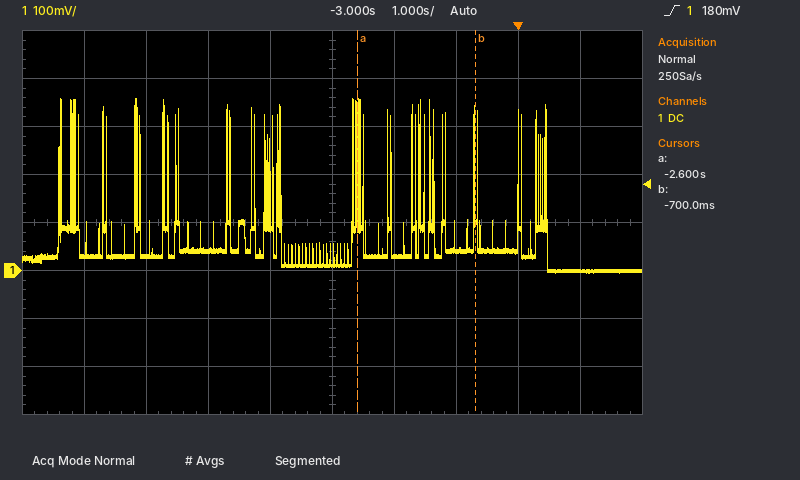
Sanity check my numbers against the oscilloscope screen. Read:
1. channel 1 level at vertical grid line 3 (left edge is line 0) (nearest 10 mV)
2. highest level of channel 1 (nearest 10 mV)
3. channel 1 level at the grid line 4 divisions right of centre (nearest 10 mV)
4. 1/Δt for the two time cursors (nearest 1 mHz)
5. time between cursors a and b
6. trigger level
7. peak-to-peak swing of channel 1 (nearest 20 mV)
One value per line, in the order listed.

40 mV
360 mV
0 mV
526 mHz
1.9 s
180 mV
360 mV
